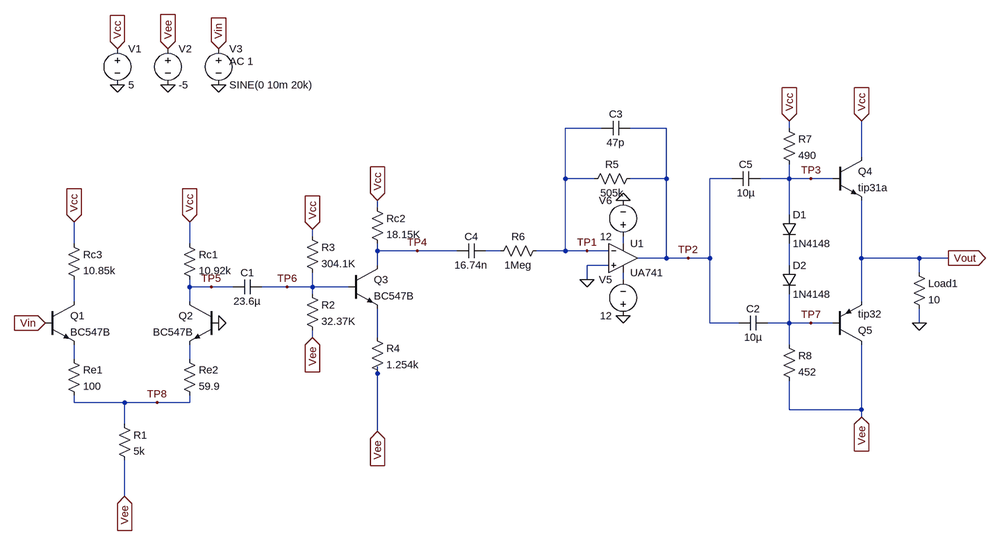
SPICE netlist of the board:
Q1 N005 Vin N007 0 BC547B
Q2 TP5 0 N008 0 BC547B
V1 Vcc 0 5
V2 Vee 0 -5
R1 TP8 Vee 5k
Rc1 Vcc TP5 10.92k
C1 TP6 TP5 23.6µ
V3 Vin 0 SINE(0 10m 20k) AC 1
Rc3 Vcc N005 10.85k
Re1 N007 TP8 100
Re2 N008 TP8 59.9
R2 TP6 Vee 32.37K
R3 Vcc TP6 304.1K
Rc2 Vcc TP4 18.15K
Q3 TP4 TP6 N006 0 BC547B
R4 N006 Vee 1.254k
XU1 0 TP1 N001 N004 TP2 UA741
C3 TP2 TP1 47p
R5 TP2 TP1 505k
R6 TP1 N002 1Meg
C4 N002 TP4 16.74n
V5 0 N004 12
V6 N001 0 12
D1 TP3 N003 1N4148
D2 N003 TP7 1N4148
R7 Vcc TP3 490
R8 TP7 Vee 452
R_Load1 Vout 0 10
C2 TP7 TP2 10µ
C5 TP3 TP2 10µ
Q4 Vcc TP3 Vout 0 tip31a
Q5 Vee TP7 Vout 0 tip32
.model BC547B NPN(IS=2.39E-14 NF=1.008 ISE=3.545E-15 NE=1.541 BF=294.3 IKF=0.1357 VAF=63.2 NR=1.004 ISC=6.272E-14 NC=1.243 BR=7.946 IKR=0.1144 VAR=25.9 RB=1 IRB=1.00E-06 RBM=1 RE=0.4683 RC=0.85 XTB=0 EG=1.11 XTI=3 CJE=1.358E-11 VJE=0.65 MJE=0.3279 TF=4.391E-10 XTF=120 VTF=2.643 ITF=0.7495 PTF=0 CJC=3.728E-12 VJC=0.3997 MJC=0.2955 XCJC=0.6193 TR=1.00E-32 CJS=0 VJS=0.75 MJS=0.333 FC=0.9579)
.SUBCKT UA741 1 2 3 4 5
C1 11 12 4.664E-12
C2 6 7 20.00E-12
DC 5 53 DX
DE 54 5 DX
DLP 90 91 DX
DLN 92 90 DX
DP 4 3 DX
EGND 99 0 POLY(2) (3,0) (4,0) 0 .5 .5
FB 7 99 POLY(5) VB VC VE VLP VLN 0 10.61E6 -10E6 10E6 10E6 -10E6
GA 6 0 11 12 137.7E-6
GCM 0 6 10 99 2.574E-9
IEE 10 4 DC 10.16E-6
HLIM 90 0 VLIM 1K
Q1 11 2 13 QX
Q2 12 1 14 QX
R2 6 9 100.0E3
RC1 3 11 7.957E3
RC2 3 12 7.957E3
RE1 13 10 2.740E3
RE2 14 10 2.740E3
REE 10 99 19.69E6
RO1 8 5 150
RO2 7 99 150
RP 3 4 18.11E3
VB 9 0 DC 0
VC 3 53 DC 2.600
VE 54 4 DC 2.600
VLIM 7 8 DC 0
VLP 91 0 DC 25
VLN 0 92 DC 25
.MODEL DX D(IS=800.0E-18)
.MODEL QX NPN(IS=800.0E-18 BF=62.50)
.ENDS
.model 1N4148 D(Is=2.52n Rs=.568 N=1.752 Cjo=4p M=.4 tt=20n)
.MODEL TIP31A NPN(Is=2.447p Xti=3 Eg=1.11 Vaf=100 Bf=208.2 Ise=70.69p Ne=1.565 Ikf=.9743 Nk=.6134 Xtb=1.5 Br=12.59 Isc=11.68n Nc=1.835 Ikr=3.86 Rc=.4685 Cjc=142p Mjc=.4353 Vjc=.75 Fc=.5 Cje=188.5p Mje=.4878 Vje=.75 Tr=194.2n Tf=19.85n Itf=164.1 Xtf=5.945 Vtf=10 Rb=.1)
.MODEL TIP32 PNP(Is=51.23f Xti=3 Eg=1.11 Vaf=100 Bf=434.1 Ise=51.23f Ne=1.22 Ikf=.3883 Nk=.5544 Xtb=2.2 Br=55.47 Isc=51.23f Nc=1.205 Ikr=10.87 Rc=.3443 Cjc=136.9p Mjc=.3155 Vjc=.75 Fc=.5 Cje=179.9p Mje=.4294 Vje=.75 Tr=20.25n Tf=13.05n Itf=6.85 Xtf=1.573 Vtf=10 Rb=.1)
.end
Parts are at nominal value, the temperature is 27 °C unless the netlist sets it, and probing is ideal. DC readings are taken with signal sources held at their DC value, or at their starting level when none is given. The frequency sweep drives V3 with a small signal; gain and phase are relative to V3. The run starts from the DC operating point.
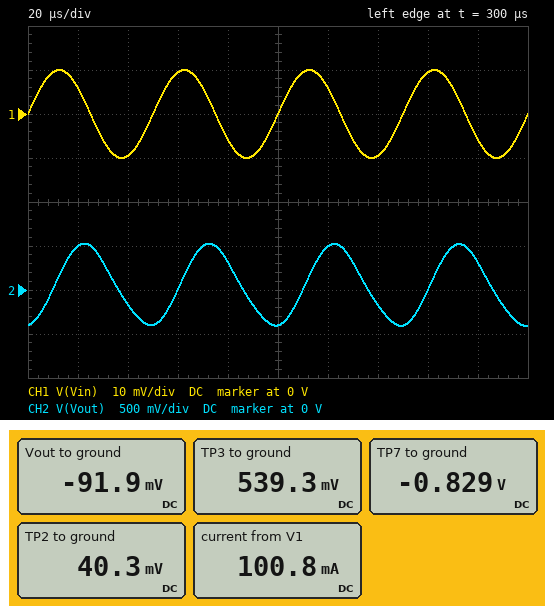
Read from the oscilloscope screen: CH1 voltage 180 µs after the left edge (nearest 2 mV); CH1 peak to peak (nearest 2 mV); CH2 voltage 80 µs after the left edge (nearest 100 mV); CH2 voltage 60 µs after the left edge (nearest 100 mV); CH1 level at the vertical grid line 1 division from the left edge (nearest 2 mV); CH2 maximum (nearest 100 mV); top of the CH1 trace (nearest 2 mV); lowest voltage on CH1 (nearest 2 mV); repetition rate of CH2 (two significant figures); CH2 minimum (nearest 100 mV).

-6 mV
20 mV
300 mV
0 V
6 mV
500 mV
10 mV
-10 mV
20 kHz
-400 mV
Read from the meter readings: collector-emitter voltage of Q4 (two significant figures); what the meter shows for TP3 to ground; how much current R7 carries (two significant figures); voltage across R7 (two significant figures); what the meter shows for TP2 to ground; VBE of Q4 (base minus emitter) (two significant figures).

5.1 V
539.3 mV
9.1 mA
4.5 V
40.3 mV
630 mV
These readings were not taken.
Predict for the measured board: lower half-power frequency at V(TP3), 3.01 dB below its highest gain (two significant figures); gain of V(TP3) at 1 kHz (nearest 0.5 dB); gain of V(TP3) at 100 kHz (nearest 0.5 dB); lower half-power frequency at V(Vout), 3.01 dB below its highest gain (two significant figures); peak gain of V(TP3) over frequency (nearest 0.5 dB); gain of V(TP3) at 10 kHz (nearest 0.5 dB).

43 Hz
44.5 dB
21.0 dB
43 Hz
44.5 dB
39.5 dB
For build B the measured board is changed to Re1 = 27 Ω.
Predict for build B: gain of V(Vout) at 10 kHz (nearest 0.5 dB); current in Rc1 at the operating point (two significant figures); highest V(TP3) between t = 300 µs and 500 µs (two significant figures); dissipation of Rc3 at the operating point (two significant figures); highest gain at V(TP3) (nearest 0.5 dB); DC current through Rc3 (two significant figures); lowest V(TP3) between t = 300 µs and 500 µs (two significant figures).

41.5 dB
370 µA
910 mV
2.7 mW
47.0 dB
500 µA
-260 mV
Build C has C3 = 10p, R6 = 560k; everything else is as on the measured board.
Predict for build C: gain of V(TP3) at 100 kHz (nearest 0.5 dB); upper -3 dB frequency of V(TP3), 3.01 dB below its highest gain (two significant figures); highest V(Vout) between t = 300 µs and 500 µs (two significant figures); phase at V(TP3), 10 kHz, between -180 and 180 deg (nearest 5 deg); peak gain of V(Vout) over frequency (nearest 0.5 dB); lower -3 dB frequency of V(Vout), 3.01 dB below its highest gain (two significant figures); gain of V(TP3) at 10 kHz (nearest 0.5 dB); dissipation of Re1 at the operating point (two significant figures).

38.5 dB
29 kHz
2.4 V
-20 deg
49.5 dB
47 Hz
49.0 dB
14 µW
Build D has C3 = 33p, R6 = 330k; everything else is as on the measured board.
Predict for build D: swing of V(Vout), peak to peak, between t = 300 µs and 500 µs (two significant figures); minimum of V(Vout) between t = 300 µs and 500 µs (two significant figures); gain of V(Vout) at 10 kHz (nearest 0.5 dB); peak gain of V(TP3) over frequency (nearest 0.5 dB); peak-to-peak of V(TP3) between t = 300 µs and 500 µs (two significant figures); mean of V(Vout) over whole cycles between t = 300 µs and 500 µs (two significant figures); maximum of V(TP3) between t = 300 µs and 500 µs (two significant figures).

3.6 V
-1.5 V
50.5 dB
54.0 dB
3.7 V
300 mV
2.8 V
